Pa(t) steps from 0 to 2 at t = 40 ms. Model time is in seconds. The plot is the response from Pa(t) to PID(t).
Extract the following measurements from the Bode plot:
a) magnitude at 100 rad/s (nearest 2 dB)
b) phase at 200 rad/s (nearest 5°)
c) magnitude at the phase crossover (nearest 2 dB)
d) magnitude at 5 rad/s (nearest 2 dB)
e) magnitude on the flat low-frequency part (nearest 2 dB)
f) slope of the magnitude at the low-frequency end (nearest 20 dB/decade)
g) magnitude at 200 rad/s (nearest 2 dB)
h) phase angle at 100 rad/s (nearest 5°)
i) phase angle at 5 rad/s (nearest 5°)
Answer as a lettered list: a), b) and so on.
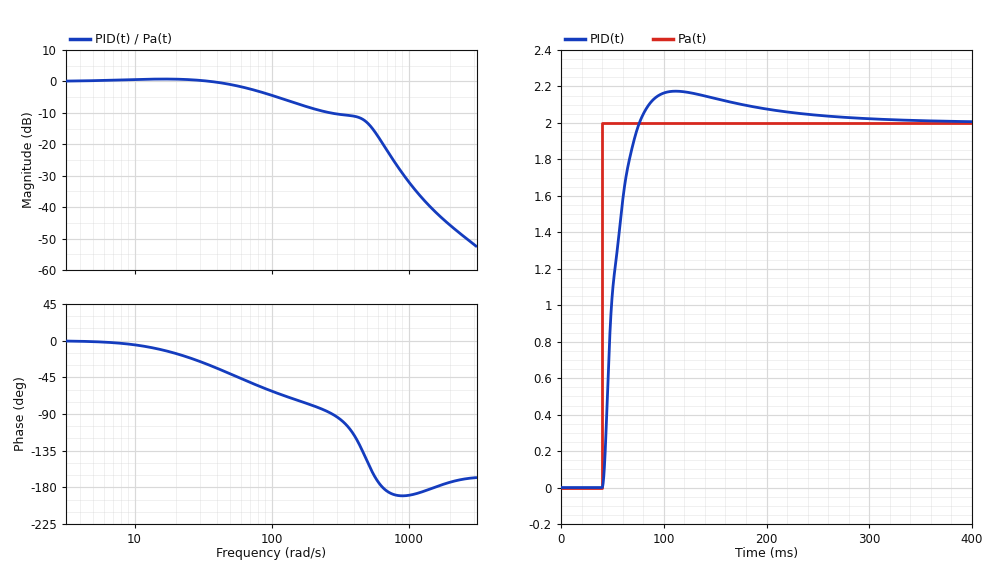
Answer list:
a) -4 dB
b) -80°
c) -20 dB
d) 0 dB
e) 0 dB
f) 0 dB/decade
g) -8 dB
h) -60°
i) 0°
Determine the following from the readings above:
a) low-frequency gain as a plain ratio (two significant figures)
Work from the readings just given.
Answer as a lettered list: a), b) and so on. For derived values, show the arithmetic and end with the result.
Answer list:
a) 10^(0 / 20) = 1.0
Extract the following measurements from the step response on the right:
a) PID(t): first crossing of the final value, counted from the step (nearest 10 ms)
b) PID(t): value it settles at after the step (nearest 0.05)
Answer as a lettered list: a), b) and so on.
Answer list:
a) 40 ms
b) 2.00
